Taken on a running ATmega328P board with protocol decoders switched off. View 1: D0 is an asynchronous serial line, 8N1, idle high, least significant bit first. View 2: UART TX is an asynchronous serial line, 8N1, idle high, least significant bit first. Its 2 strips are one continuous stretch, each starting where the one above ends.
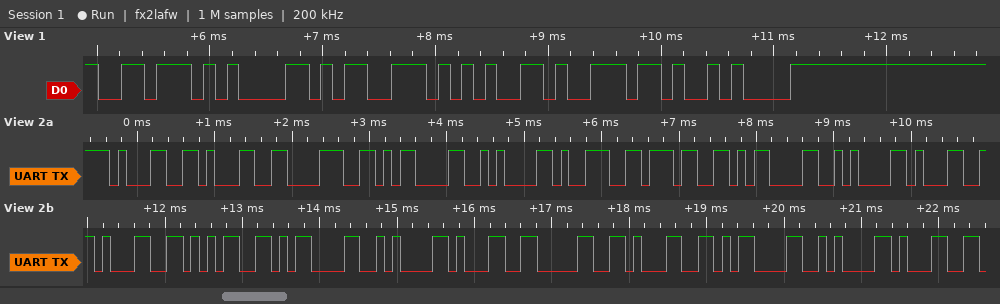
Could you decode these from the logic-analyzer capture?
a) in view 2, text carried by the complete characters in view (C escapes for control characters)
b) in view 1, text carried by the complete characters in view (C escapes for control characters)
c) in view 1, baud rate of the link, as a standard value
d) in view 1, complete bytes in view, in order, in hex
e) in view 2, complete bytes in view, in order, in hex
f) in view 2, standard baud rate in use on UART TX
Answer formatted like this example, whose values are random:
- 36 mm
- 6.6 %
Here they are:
- "118\r\n97\r\n115\r\n101\r\n1"
- "vasen\n"
- 9600 baud
- 76 61 73 65 6E 0A
- 31 31 38 0D 0A 39 37 0D 0A 31 31 35 0D 0A 31 30 31 0D 0A 31
- 9600 baud
